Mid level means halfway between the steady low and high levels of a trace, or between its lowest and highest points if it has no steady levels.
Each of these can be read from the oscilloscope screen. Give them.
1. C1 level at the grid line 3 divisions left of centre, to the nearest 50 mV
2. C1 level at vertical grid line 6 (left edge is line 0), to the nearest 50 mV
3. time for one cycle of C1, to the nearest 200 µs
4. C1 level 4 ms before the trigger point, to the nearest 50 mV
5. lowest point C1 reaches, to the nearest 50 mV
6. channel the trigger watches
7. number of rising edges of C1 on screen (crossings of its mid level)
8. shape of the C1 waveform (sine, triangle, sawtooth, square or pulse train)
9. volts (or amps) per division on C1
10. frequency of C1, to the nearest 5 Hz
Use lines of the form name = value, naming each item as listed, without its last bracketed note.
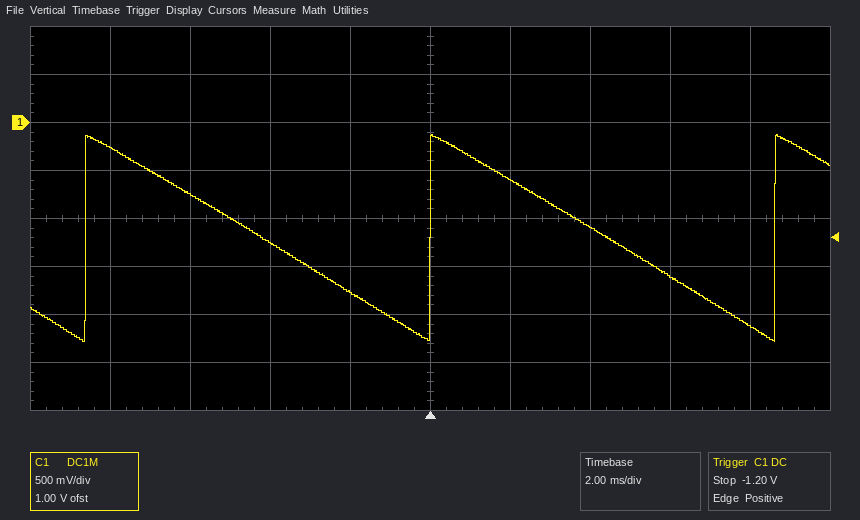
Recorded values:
C1 level at the grid line 3 divisions left of centre, to the nearest 50 mV = -750 mV
C1 level at vertical grid line 6 (left edge is line 0), to the nearest 50 mV = -600 mV
time for one cycle of C1, to the nearest 200 µs = 8.6 ms
C1 level 4 ms before the trigger point, to the nearest 50 mV = -1.25 V
lowest point C1 reaches, to the nearest 50 mV = -2.30 V
channel the trigger watches = C1
number of rising edges of C1 on screen = 3
shape of the C1 waveform = sawtooth
volts (or amps) per division on C1 = 500 mV
frequency of C1, to the nearest 5 Hz = 115 Hz
